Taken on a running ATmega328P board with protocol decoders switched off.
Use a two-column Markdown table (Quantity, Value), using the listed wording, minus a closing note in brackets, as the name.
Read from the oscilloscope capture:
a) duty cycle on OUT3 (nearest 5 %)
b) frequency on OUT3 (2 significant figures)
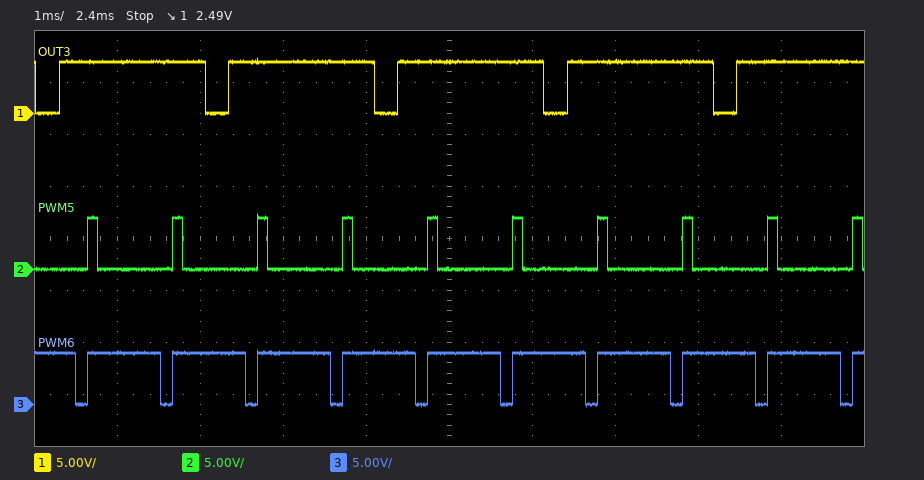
| Quantity | Value |
|---|---|
| duty cycle on OUT3 | 85 % |
| frequency on OUT3 | 490 Hz |
